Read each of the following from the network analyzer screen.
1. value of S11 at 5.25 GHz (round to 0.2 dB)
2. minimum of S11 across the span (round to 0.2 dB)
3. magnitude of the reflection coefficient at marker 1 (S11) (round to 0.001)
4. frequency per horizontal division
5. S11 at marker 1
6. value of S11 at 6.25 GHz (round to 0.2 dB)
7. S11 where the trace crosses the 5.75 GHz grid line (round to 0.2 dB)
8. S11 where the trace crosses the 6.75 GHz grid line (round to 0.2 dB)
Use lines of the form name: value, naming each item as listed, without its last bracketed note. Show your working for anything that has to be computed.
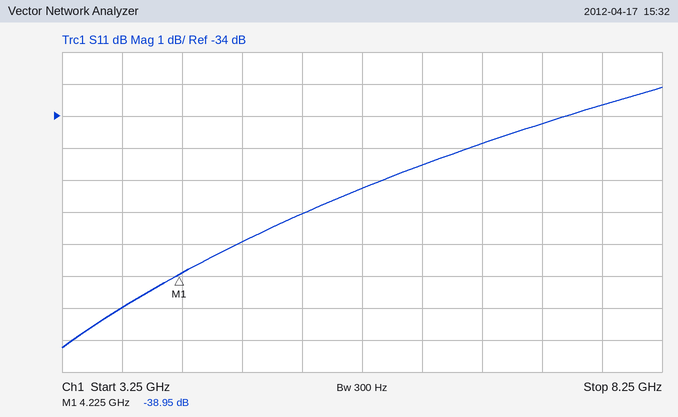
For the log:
value of S11 at 5.25 GHz: -37.0 dB
minimum of S11 across the span: -41.2 dB
magnitude of the reflection coefficient at marker 1 (S11): 10^(-38.95/20) ≈ 0.011
frequency per horizontal division: 500 MHz
S11 at marker 1: -38.95 dB
value of S11 at 6.25 GHz: -35.6 dB
S11 where the trace crosses the 5.75 GHz grid line: -36.2 dB
S11 where the trace crosses the 6.75 GHz grid line: -34.8 dB
